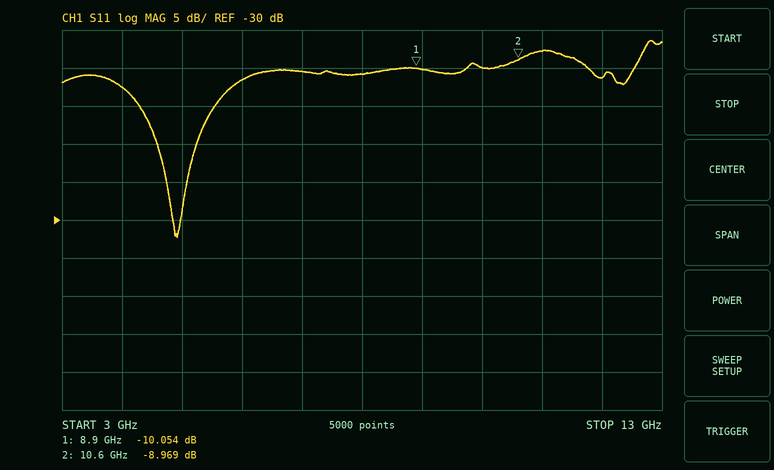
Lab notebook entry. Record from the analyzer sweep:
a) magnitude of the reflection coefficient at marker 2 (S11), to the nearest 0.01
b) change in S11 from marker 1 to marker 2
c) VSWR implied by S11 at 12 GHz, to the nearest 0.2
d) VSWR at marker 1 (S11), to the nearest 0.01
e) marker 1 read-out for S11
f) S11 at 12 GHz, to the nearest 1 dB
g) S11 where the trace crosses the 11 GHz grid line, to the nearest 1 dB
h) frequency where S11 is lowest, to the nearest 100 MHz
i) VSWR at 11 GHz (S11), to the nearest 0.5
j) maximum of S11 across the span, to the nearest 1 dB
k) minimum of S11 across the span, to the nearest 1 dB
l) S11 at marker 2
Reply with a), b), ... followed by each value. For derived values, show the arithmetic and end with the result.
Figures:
a) 10^(-8.969/20) ≈ 0.36
b) -8.969 − (-10.054) = 1.085 dB
c) |Γ| = 10^(-11/20) = 0.2818; VSWR = (1 + 0.2818)/(1 − 0.2818) ≈ 1.8
d) (1 + 0.3143)/(1 − 0.3143) ≈ 1.92
e) -10.054 dB
f) -11 dB
g) -8 dB
h) 4.9 GHz
i) |Γ| = 10^(-8/20) = 0.3981; VSWR = (1 + 0.3981)/(1 − 0.3981) ≈ 2.32, so 2.5 to the nearest 0.5
j) -6 dB
k) -32 dB
l) -8.969 dB
